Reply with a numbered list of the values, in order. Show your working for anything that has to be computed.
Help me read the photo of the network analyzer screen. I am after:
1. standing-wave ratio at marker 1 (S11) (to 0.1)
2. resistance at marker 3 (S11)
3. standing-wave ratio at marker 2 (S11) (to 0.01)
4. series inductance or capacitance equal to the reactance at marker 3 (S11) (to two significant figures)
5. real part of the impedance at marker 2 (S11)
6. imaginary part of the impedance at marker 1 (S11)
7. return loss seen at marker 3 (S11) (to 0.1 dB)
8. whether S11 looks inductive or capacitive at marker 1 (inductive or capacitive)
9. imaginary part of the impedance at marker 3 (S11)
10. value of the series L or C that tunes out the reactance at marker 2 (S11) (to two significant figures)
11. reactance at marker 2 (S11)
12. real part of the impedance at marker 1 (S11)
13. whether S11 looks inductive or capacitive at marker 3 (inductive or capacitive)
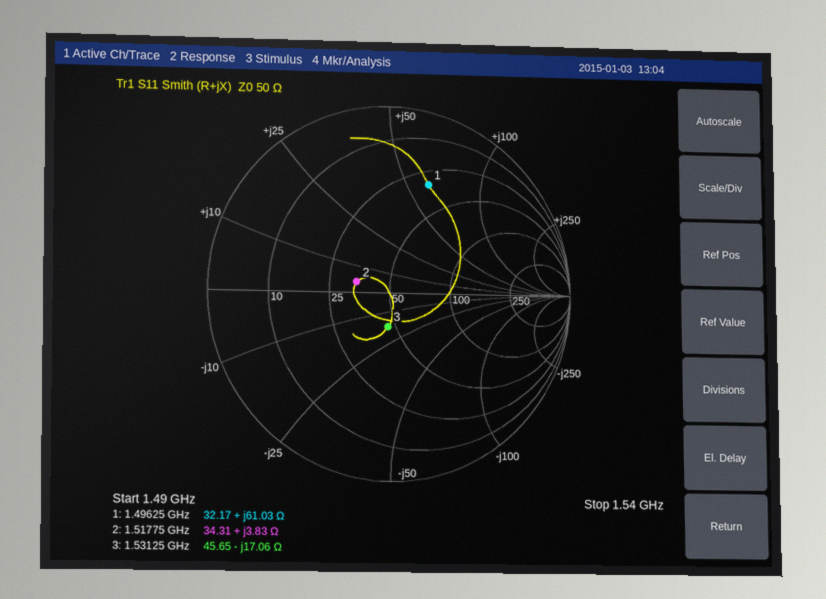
1. 4.3
2. 45.65 Ω
3. 1.47
4. C = 1/(2π × 1.53125 GHz × 17.06 Ω) ≈ 6.1 pF
5. 34.31 Ω
6. +61.03 Ω
7. 14.8 dB
8. inductive
9. -17.06 Ω
10. C = 1/(2π × 1.51775 GHz × 3.83 Ω) ≈ 27 pF
11. +3.83 Ω
12. 32.17 Ω
13. capacitive
